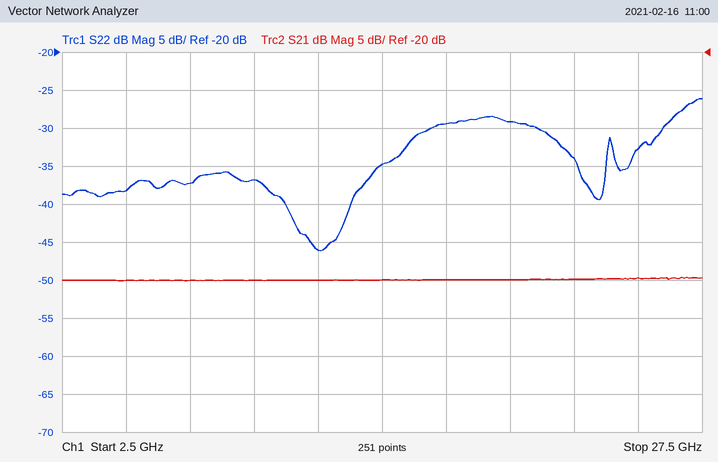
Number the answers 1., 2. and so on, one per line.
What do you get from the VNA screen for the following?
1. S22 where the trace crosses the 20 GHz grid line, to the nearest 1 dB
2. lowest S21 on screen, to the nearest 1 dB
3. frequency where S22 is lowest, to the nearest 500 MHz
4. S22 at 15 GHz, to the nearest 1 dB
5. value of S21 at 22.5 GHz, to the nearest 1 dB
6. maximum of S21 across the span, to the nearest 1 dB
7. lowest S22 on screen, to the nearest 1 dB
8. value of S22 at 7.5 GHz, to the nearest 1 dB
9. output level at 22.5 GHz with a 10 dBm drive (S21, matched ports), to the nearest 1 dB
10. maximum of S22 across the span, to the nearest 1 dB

1. -29 dB
2. -50 dB
3. 12.5 GHz
4. -35 dB
5. -50 dB
6. -50 dB
7. -46 dB
8. -37 dB
9. -40 dBm
10. -26 dB
